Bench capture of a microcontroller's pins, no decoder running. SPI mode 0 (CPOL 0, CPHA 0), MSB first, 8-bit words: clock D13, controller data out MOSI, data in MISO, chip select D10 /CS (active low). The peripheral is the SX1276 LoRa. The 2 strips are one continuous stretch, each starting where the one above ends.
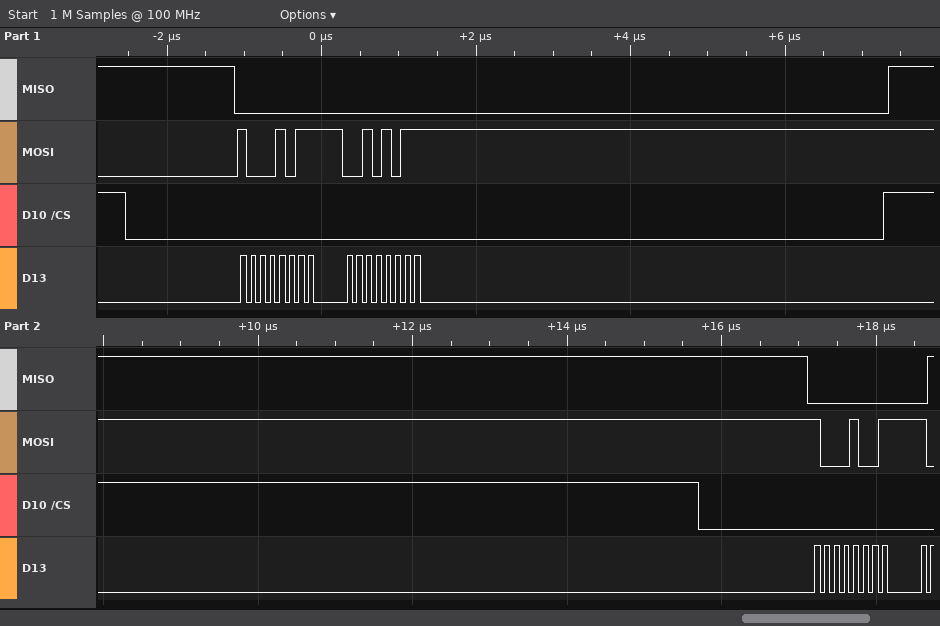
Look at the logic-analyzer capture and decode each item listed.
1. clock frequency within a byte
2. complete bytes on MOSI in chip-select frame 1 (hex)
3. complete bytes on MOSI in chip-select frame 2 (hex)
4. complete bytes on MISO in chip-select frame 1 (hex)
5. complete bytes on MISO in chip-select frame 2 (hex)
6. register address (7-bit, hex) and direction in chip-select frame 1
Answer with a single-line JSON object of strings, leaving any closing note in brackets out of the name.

{"clock frequency within a byte": "8 MHz", "complete bytes on MOSI in chip-select frame 1": "8B 2B", "complete bytes on MOSI in chip-select frame 2": "89", "complete bytes on MISO in chip-select frame 1": "00 00", "complete bytes on MISO in chip-select frame 2": "00", "register address (7-bit, hex) and direction in chip-select frame 1": "0x0B write"}
